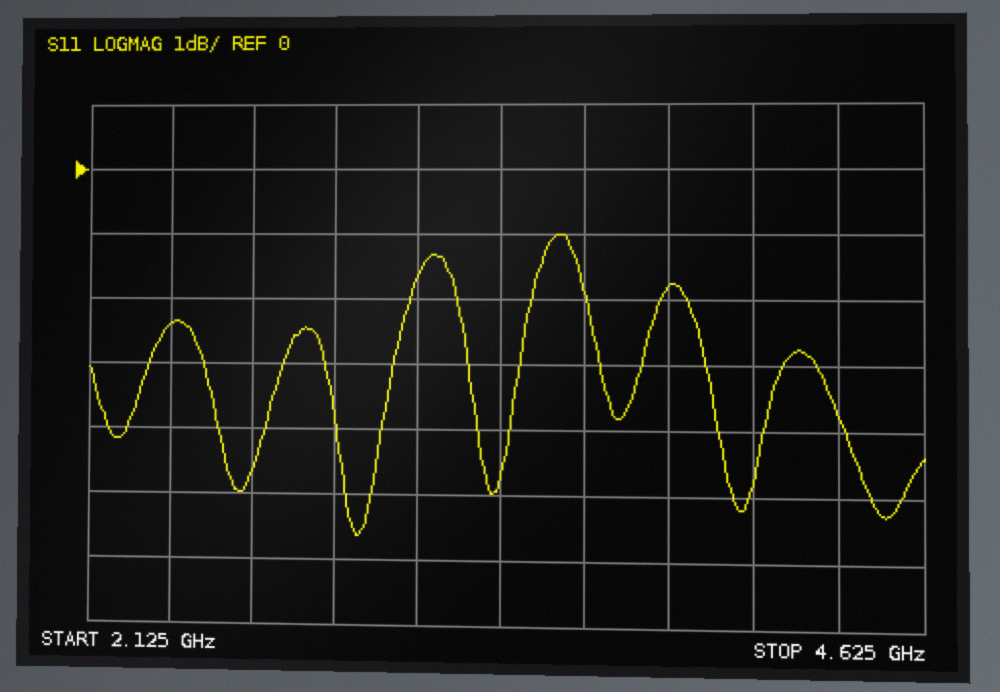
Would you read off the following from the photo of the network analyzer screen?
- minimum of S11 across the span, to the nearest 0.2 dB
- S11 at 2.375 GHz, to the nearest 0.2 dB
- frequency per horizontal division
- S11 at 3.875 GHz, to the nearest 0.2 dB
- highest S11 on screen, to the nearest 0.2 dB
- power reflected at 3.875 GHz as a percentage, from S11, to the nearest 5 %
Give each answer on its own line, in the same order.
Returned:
-5.6 dB
-2.4 dB
250 MHz
-1.8 dB
-1.0 dB
65 %
